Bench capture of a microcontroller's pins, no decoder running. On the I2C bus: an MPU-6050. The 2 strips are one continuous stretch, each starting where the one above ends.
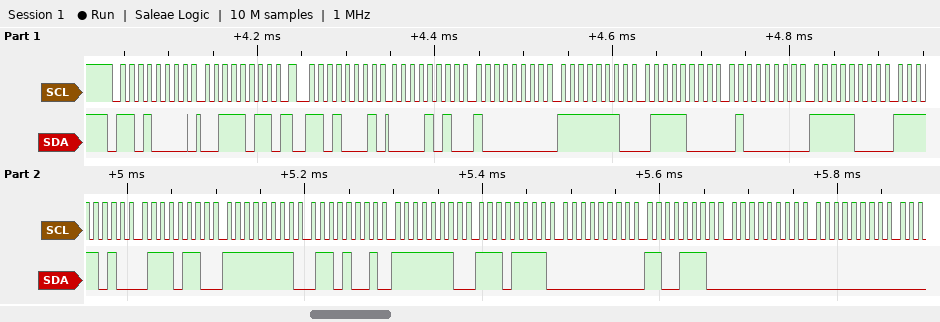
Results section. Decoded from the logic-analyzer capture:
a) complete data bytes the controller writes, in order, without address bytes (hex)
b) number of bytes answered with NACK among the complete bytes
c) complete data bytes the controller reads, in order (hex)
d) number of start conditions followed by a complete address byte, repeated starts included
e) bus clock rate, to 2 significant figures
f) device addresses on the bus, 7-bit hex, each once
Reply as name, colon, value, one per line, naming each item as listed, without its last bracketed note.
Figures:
complete data bytes the controller writes, in order, without address bytes: 3B
number of bytes answered with NACK among the complete bytes: 0
complete data bytes the controller reads, in order: 0A 80 FE 78 40 F8 FA 76 FF 69 FE EF 00 CE 00 00
number of start conditions followed by a complete address byte, repeated starts included: 2
bus clock rate, to 2 significant figures: 100 kHz
device addresses on the bus, 7-bit hex, each once: 0x68
